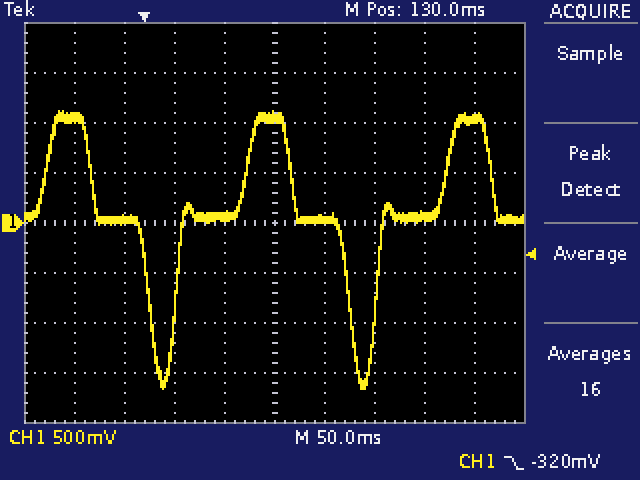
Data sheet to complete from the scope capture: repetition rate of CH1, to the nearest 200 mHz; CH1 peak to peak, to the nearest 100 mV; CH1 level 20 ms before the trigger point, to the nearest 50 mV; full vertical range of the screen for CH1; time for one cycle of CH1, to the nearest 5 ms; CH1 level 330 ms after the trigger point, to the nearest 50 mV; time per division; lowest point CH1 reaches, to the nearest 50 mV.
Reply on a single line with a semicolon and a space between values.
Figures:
5.0 Hz; 2.80 V; 50 mV; 4 V; 200 ms; 1.05 V; 50 ms; -1.65 V
